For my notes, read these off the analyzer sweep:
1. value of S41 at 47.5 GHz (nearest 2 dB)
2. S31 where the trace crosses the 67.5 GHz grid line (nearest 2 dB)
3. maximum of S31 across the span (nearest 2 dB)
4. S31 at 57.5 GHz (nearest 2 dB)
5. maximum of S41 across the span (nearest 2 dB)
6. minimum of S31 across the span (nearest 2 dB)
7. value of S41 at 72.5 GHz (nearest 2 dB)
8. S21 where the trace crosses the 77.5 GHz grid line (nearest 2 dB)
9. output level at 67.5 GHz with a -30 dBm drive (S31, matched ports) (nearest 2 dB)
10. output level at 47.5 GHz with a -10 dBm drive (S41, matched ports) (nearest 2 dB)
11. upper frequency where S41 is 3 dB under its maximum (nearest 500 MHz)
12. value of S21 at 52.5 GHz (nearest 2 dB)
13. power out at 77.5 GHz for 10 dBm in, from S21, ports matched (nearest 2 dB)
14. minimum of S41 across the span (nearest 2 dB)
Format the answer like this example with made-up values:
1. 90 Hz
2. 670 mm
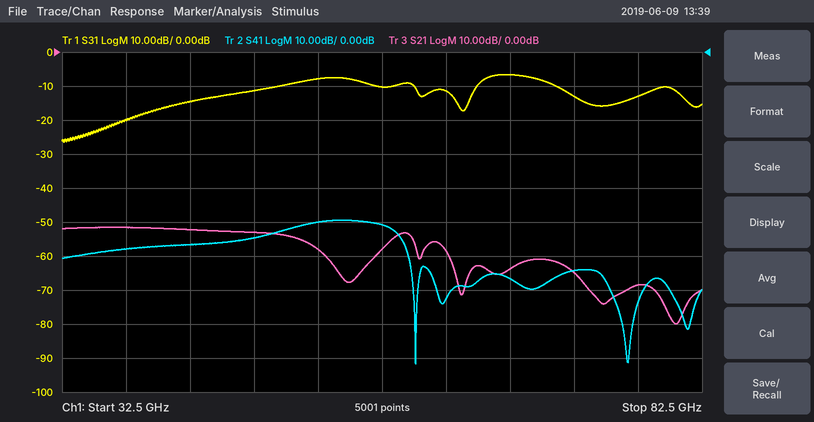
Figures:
1. -54 dB
2. -6 dB
3. -6 dB
4. -10 dB
5. -50 dB
6. -26 dB
7. -64 dB
8. -68 dB
9. -36 dBm
10. -64 dBm
11. 58.5 GHz
12. -58 dB
13. -58 dBm
14. -92 dB
